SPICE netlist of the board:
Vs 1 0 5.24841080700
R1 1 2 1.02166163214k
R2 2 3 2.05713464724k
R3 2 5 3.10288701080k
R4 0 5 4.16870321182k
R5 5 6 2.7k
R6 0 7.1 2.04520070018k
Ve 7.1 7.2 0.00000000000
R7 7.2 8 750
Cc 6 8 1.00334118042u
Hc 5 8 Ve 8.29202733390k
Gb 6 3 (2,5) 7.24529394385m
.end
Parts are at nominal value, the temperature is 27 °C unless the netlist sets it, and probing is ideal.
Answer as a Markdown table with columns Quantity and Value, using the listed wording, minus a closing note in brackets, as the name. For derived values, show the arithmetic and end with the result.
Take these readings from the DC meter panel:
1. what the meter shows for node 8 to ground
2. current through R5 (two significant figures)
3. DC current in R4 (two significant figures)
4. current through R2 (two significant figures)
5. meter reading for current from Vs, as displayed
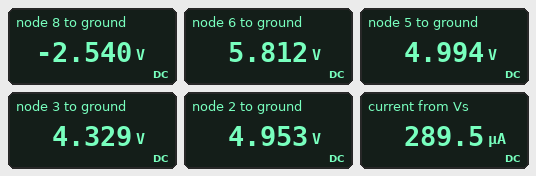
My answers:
| Quantity | Value |
|---|---|
| what the meter shows for node 8 to ground | -2.540 V |
| current through R5 | (5.812 V - 4.994 V) / 2.7 kΩ = 300 µA |
| DC current in R4 | (4.994 V) / 4.169 kΩ = 1.2 mA |
| current through R2 | (4.953 V - 4.329 V) / 2.057 kΩ = 300 µA |
| meter reading for current from Vs, as displayed | 289.5 µA |
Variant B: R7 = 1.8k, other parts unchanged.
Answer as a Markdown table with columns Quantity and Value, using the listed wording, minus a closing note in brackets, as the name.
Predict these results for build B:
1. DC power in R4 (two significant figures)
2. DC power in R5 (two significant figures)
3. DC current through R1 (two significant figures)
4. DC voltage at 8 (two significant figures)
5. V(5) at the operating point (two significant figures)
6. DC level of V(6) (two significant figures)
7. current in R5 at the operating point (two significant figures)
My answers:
| Quantity | Value |
|---|---|
| DC power in R4 | 6.4 mW |
| DC power in R5 | 18 µW |
| DC current through R1 | 78 µA |
| DC voltage at 8 | -4.5 V |
| V(5) at the operating point | 5.2 V |
| DC level of V(6) | 5.4 V |
| current in R5 at the operating point | 81 µA |
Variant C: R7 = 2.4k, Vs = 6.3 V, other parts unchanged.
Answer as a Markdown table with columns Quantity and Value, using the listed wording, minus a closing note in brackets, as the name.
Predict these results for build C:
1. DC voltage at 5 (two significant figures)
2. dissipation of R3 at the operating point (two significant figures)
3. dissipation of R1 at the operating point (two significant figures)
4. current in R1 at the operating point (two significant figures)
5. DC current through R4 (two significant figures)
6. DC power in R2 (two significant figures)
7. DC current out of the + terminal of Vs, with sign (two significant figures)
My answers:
| Quantity | Value |
|---|---|
| DC voltage at 5 | 6.4 V |
| dissipation of R3 at the operating point | 110 nW |
| dissipation of R1 at the operating point | 17 µW |
| current in R1 at the operating point | 130 µA |
| DC current through R4 | 1.5 mA |
| DC power in R2 | 37 µW |
| DC current out of the + terminal of Vs, with sign | -130 µA |
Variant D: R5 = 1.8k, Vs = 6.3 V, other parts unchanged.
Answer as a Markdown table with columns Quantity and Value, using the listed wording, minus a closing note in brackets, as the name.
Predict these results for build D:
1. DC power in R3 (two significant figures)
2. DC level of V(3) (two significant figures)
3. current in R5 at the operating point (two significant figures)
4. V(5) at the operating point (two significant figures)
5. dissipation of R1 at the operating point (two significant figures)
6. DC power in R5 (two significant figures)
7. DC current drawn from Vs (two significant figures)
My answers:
| Quantity | Value |
|---|---|
| DC power in R3 | 810 nW |
| DC level of V(3) | 5.2 V |
| current in R5 at the operating point | 360 µA |
| V(5) at the operating point | 6.0 V |
| dissipation of R1 at the operating point | 120 µW |
| DC power in R5 | 240 µW |
| DC current drawn from Vs | 350 µA |
